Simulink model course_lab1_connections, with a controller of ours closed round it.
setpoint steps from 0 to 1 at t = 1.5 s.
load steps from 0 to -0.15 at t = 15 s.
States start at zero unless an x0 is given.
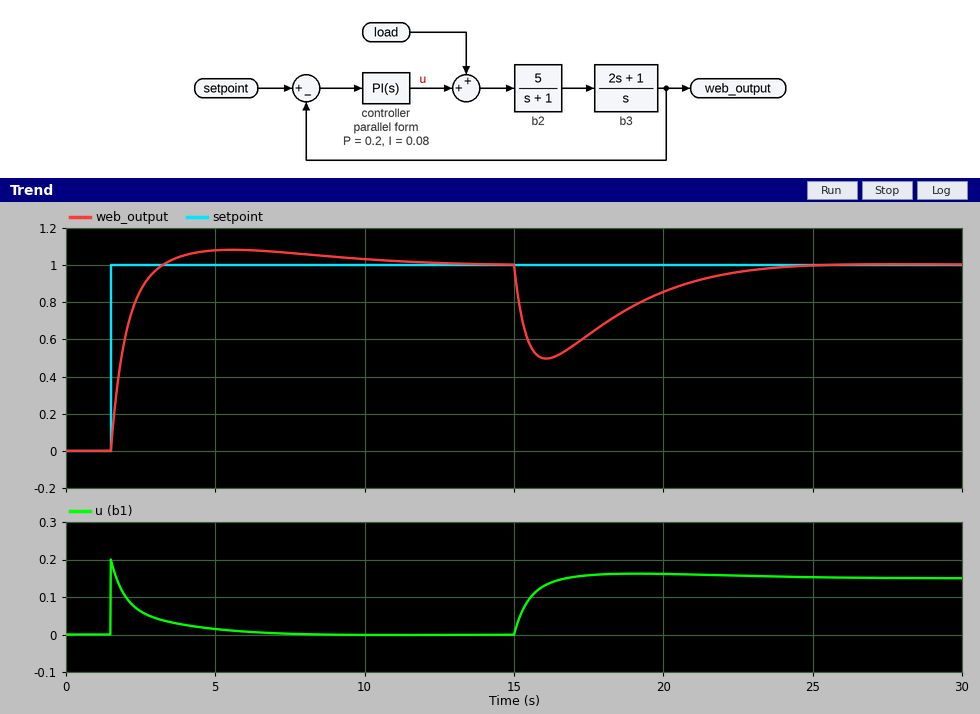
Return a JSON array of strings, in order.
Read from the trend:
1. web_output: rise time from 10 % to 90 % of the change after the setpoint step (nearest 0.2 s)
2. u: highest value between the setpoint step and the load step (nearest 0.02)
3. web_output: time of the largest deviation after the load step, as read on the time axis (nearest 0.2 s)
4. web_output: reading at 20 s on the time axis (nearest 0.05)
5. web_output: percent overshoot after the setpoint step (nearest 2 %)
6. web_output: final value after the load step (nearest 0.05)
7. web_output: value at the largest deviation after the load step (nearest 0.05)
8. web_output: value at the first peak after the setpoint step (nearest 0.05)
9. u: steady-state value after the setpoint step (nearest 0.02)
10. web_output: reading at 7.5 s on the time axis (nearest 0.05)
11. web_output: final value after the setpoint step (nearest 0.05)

["1.0 s", "0.20", "16.0 s", "0.85", "8 %", "1.00", "0.50", "1.10", "0.00", "1.05", "1.00"]
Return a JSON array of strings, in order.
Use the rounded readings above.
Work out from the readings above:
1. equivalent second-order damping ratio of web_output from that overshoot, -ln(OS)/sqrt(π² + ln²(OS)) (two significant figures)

["0.63"]
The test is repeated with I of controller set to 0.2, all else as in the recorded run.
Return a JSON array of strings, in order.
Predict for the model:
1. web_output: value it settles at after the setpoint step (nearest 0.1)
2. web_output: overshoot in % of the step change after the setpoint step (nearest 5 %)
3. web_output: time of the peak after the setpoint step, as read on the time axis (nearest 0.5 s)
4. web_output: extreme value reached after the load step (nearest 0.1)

["1.0", "15 %", "3.5 s", "0.6"]
